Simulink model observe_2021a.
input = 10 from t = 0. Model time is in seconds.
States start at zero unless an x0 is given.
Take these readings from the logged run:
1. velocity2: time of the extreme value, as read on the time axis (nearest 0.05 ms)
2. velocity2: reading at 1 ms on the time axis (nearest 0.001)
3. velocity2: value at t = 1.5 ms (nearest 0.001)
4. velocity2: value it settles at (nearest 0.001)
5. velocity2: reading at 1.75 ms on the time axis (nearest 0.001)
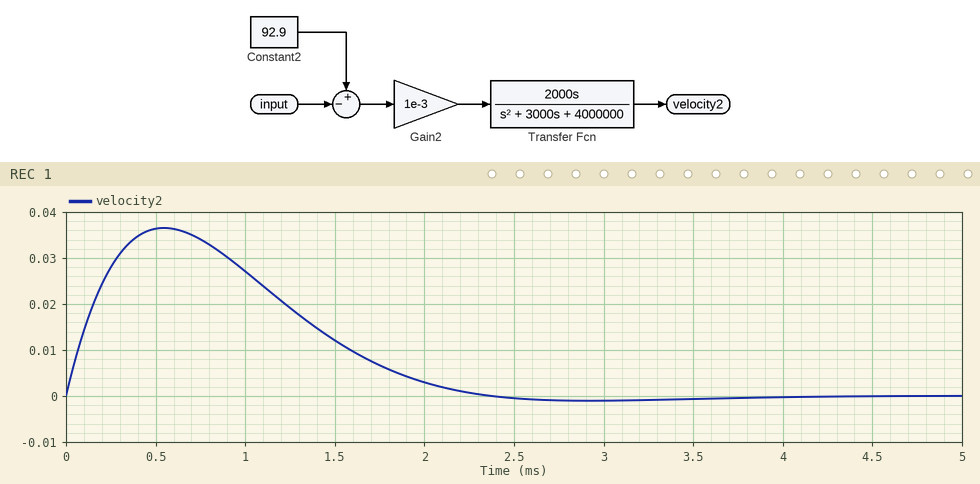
0.55 ms
0.027
0.012
0.000
0.007
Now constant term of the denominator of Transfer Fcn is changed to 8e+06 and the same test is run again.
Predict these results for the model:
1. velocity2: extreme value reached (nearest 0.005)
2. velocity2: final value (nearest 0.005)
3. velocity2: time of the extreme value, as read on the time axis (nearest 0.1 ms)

0.030
0.000
0.4 ms
